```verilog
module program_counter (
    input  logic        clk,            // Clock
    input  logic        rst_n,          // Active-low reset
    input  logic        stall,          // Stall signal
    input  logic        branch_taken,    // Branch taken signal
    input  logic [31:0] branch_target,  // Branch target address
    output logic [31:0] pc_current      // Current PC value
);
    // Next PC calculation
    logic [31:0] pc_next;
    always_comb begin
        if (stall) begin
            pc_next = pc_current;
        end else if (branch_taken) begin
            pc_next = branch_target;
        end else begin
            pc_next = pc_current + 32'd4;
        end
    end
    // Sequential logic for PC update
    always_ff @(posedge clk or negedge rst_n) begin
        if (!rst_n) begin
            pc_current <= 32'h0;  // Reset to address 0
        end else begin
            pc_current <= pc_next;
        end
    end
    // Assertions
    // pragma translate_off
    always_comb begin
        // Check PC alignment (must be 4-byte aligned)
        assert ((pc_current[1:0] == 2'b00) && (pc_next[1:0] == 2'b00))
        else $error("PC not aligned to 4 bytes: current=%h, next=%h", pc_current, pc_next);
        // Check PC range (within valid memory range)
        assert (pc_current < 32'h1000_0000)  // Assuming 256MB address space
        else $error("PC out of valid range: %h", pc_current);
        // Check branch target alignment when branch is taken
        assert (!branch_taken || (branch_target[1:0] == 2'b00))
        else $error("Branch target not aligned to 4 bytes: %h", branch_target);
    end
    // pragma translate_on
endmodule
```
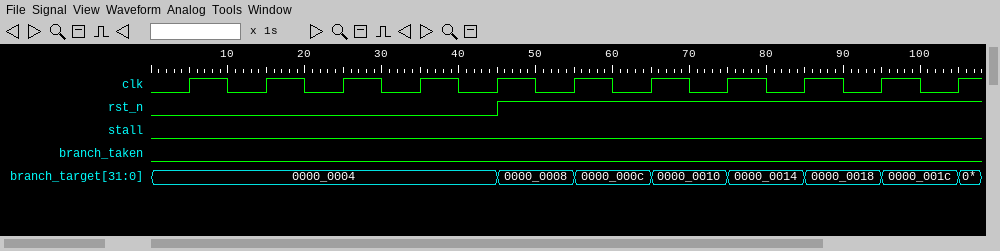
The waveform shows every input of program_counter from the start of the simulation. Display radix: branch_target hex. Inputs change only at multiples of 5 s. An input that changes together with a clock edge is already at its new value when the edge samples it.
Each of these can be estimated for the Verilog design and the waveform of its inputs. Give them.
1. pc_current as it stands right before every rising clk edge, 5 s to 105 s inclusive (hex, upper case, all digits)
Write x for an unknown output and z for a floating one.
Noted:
00000000, 00000000, 00000000, 00000000, 00000000, 00000004, 00000008, 0000000C, 00000010, 00000014, 00000018
